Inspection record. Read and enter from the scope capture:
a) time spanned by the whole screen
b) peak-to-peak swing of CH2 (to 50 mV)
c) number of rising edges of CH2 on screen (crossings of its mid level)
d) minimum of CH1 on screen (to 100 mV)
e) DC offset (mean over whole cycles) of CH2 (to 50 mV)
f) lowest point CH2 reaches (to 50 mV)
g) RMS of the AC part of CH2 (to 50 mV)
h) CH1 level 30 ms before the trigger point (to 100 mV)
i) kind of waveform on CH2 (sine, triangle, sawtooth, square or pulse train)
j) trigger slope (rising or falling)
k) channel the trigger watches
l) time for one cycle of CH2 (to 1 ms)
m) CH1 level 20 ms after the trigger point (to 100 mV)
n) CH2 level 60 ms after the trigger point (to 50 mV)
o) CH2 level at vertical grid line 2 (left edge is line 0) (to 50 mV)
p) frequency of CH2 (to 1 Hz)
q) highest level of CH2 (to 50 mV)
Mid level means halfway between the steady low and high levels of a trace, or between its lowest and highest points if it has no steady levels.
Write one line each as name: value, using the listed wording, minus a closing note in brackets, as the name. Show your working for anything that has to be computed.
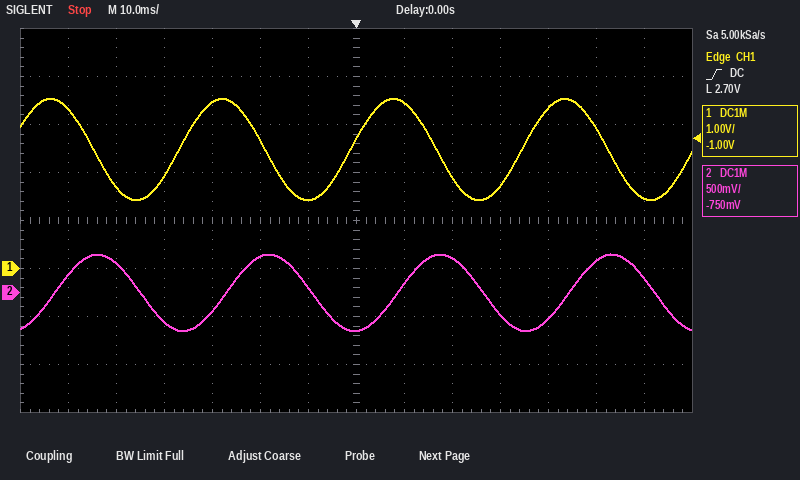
time spanned by the whole screen: 140 ms
peak-to-peak swing of CH2: 400 mV − (-400 mV) = 800 mV
number of rising edges of CH2 on screen: 4
minimum of CH1 on screen: 1.4 V
DC offset (mean over whole cycles) of CH2: (400 mV + (-400 mV)) / 2 ≈ 0 mV
lowest point CH2 reaches: -400 mV
RMS of the AC part of CH2: 800 mV / (2√2) ≈ 283 mV, so 300 mV to the nearest 50 mV
CH1 level 30 ms before the trigger point: 3.5 V
kind of waveform on CH2: sine
trigger slope: rising
channel the trigger watches: CH1
time for one cycle of CH2: 36 ms
CH1 level 20 ms after the trigger point: 1.9 V
CH2 level 60 ms after the trigger point: 150 mV
CH2 level at vertical grid line 2 (left edge is line 0): 300 mV
frequency of CH2: 1 / 36 ms ≈ 28 Hz
highest level of CH2: 400 mV
